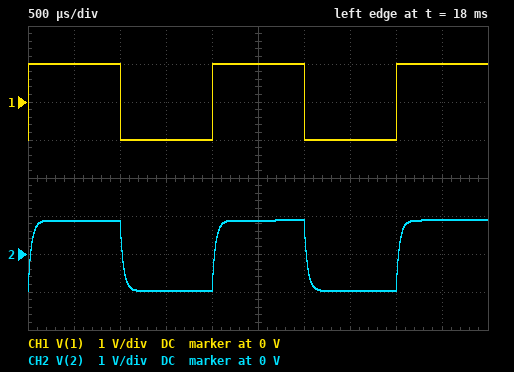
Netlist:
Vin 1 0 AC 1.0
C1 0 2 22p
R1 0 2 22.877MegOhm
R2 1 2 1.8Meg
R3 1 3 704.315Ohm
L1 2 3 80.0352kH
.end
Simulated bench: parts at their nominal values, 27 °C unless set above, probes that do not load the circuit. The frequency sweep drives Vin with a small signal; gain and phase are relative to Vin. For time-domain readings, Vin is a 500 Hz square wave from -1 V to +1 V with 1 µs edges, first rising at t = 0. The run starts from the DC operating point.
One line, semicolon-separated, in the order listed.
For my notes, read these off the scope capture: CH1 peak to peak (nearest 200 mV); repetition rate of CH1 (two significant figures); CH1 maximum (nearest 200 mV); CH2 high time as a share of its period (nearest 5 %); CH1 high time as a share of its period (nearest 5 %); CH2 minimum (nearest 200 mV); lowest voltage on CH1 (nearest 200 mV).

2.0 V; 500 Hz; 1.0 V; 50 %; 50 %; -1.0 V; -1.0 V
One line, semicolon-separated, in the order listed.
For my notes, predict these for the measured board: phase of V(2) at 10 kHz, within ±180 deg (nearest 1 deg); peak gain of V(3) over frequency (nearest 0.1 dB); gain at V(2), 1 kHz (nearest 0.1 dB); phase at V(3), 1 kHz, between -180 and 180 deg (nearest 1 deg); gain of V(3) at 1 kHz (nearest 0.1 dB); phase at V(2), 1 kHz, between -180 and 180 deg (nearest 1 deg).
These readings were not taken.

-67 deg; 0 dB; -0.9 dB; 0 deg; 0 dB; -13 deg
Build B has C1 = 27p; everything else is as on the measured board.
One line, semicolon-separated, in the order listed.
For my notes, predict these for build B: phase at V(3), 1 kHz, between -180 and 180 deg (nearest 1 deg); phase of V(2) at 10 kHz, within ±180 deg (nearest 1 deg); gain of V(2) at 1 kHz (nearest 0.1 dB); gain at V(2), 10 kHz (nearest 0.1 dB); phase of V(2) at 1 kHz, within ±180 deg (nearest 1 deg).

0 deg; -71 deg; -1.0 dB; -10.2 dB; -16 deg
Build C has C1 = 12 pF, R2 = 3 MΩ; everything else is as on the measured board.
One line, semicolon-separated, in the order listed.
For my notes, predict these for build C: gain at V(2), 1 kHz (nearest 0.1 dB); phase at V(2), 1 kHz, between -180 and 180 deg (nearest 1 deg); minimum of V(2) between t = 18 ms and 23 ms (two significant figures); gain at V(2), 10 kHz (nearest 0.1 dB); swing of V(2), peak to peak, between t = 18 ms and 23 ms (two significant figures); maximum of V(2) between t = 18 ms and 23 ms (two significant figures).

-1.2 dB; -11 deg; -950 mV; -8.1 dB; 1.8 V; 830 mV
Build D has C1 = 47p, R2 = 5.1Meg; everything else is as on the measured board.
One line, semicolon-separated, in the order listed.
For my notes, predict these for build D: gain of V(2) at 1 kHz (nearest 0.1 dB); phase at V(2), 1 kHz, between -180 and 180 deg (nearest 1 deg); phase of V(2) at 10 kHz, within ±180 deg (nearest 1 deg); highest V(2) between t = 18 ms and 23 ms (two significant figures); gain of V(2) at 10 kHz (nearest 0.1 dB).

-5.7 dB; -51 deg; -85 deg; 770 mV; -23.6 dB
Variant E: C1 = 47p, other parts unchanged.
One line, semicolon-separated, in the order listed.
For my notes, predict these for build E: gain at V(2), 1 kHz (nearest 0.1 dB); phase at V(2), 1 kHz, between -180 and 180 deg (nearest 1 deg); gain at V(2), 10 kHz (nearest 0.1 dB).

-1.6 dB; -26 deg; -14.7 dB
